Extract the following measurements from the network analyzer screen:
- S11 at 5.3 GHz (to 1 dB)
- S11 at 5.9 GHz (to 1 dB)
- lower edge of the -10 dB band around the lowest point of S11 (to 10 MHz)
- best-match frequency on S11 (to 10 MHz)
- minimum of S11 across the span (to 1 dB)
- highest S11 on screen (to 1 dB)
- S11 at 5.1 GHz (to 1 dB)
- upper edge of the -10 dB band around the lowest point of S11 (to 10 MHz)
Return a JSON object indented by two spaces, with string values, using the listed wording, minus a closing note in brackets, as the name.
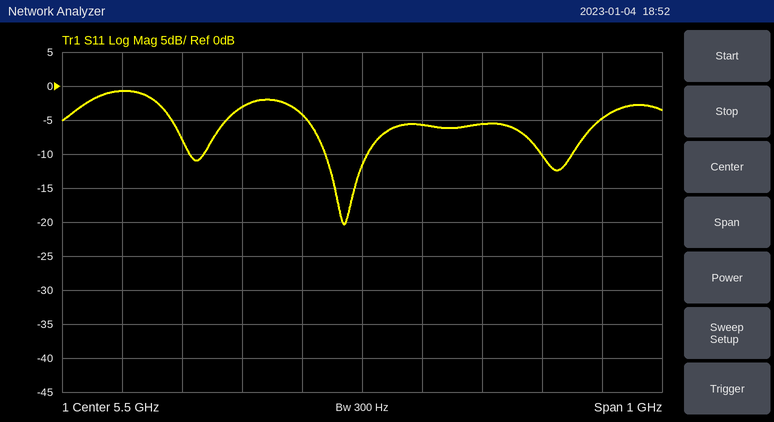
{
  "S11 at 5.3 GHz": "-3 dB",
  "S11 at 5.9 GHz": "-5 dB",
  "lower edge of the -10 dB band around the lowest point of S11": "5.44 GHz",
  "best-match frequency on S11": "5.47 GHz",
  "minimum of S11 across the span": "-20 dB",
  "highest S11 on screen": "-1 dB",
  "S11 at 5.1 GHz": "-1 dB",
  "upper edge of the -10 dB band around the lowest point of S11": "5.51 GHz"
}
